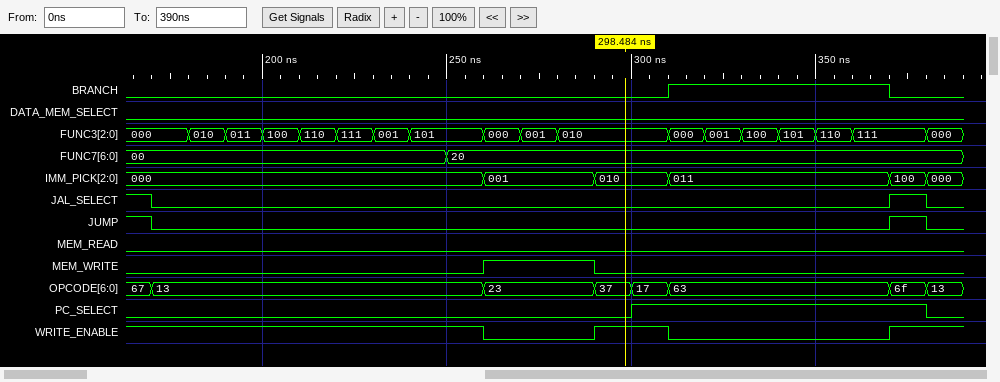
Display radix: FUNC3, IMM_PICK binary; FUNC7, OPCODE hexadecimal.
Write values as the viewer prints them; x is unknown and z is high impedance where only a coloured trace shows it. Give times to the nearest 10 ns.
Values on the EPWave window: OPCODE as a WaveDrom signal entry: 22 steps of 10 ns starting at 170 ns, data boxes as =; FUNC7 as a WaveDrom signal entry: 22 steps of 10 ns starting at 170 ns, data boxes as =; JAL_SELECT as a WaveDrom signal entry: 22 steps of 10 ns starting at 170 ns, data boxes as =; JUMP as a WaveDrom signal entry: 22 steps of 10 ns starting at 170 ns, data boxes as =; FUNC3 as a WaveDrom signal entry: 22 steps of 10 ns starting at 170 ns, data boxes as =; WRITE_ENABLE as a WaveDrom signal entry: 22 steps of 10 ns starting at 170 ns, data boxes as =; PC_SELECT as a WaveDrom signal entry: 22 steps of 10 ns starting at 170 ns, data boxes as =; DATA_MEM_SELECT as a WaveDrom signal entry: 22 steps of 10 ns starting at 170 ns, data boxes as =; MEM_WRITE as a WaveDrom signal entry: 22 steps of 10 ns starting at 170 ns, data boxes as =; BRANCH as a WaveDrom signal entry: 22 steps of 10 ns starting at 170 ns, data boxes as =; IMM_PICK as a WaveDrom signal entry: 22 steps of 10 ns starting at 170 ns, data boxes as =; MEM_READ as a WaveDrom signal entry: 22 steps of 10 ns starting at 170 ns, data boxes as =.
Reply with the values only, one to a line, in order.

{name: 'OPCODE', wave: '=........=..===.....==', data: '13 23 37 17 63 6f 13'}
{name: 'FUNC7', wave: '=.......=.............', data: '00 20'}
{name: 'JAL_SELECT', wave: '0...................10'}
{name: 'JUMP', wave: '0...................10'}
{name: 'FUNC3', wave: '========.===..======.=', data: '000 010 011 100 110 111 001 101 000 001 010 000 001 100 101 110 111 000'}
{name: 'WRITE_ENABLE', wave: '1........0..1.0.....1.'}
{name: 'PC_SELECT', wave: '0............1.......0'}
{name: 'DATA_MEM_SELECT', wave: '0.....................'}
{name: 'MEM_WRITE', wave: '0........1..0.........'}
{name: 'BRANCH', wave: '0.............1.....0.'}
{name: 'IMM_PICK', wave: '=........=..=.=.....==', data: '000 001 010 011 100 000'}
{name: 'MEM_READ', wave: '0.....................'}
